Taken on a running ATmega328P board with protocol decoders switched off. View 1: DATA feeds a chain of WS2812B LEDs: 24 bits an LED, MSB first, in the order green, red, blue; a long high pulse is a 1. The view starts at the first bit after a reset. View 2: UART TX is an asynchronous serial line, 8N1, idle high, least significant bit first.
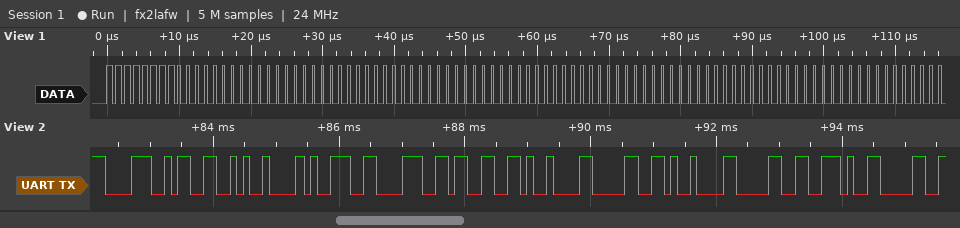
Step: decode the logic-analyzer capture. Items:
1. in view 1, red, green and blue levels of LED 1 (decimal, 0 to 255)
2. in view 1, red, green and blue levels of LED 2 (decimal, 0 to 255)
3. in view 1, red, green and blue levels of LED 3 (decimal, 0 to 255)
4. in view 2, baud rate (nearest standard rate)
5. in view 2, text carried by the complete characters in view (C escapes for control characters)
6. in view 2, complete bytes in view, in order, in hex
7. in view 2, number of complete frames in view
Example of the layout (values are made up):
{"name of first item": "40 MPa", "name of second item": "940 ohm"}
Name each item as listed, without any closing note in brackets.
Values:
{"in view 1, red, green and blue levels of LED 1": "0, 255, 0", "in view 1, red, green and blue levels of LED 2": "0, 0, 0", "in view 1, red, green and blue levels of LED 3": "0, 0, 0", "in view 2, baud rate": "9600 baud", "in view 2, text carried by the complete characters in view": "\"83\\t983\\t0\\t0.0\"", "in view 2, complete bytes in view, in order, in hex": "0x38 0x33 0x09 0x39 0x38 0x33 0x09 0x30 0x09 0x30 0x2E 0x30", "in view 2, number of complete frames in view": "12"}
